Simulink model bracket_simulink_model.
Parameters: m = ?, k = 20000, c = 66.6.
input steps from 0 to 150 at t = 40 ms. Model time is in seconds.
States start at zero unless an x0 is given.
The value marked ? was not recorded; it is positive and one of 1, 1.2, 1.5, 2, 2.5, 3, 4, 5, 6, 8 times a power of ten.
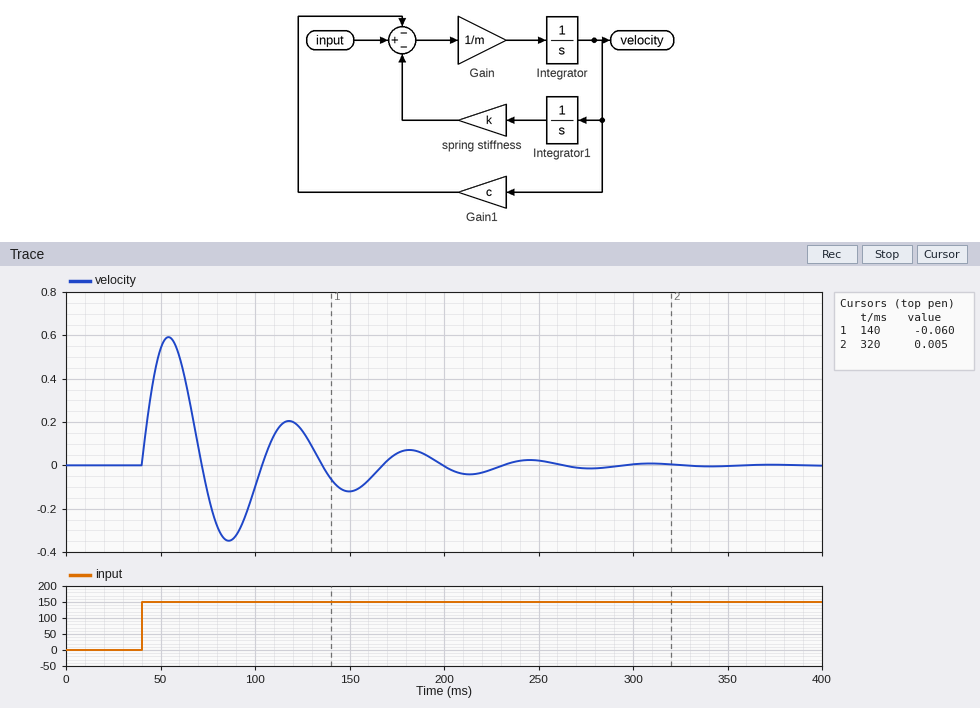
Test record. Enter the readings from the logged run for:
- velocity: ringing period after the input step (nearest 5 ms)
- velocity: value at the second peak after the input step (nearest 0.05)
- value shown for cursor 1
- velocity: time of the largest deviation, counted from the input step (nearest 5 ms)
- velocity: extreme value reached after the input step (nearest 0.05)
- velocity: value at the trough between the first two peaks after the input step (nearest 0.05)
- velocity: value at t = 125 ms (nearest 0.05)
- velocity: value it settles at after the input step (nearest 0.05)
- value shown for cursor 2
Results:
65 ms
0.20
-0.060
15 ms
0.60
-0.35
0.15
0.00
0.005
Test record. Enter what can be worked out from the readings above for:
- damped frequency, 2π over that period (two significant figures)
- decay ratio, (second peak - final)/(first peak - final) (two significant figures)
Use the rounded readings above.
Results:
0.097 rad/ms
0.33
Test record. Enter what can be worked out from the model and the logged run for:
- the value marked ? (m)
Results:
2
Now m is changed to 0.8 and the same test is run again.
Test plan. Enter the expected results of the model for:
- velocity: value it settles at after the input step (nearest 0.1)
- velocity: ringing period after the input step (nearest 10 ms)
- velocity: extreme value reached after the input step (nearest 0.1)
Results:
0.0
40 ms
0.8
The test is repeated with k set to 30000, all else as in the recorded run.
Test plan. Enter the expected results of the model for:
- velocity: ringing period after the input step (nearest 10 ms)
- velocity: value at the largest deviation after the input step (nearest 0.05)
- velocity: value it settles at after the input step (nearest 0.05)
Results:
50 ms
0.50
0.00
